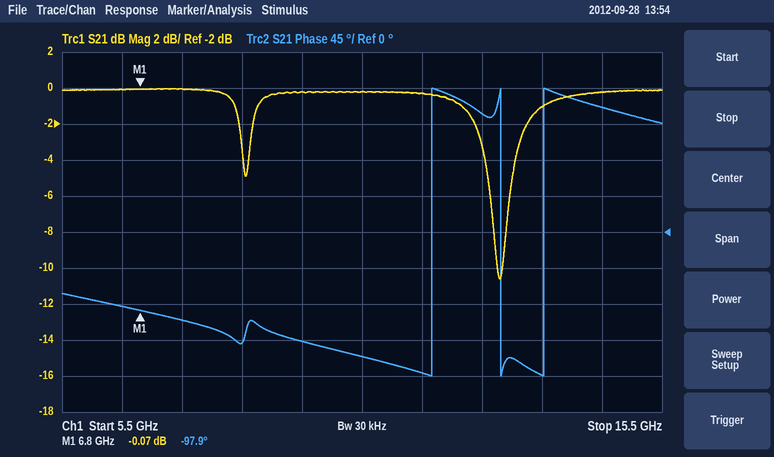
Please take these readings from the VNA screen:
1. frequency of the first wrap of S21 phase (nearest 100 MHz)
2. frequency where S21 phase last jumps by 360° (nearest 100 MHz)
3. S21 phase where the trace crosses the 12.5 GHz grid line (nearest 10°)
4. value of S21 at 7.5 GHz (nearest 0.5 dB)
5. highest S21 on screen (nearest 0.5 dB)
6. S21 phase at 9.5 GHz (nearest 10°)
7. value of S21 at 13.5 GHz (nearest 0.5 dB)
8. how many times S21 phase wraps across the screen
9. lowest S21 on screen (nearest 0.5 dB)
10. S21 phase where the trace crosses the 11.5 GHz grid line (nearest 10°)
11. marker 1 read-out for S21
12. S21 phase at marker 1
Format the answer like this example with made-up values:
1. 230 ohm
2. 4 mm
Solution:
1. 11.7 GHz
2. 13.5 GHz
3. 150°
4. 0.0 dB
5. 0.0 dB
6. -140°
7. -1.0 dB
8. 3
9. -10.5 dB
10. -180°
11. -0.07 dB
12. -97.9°
